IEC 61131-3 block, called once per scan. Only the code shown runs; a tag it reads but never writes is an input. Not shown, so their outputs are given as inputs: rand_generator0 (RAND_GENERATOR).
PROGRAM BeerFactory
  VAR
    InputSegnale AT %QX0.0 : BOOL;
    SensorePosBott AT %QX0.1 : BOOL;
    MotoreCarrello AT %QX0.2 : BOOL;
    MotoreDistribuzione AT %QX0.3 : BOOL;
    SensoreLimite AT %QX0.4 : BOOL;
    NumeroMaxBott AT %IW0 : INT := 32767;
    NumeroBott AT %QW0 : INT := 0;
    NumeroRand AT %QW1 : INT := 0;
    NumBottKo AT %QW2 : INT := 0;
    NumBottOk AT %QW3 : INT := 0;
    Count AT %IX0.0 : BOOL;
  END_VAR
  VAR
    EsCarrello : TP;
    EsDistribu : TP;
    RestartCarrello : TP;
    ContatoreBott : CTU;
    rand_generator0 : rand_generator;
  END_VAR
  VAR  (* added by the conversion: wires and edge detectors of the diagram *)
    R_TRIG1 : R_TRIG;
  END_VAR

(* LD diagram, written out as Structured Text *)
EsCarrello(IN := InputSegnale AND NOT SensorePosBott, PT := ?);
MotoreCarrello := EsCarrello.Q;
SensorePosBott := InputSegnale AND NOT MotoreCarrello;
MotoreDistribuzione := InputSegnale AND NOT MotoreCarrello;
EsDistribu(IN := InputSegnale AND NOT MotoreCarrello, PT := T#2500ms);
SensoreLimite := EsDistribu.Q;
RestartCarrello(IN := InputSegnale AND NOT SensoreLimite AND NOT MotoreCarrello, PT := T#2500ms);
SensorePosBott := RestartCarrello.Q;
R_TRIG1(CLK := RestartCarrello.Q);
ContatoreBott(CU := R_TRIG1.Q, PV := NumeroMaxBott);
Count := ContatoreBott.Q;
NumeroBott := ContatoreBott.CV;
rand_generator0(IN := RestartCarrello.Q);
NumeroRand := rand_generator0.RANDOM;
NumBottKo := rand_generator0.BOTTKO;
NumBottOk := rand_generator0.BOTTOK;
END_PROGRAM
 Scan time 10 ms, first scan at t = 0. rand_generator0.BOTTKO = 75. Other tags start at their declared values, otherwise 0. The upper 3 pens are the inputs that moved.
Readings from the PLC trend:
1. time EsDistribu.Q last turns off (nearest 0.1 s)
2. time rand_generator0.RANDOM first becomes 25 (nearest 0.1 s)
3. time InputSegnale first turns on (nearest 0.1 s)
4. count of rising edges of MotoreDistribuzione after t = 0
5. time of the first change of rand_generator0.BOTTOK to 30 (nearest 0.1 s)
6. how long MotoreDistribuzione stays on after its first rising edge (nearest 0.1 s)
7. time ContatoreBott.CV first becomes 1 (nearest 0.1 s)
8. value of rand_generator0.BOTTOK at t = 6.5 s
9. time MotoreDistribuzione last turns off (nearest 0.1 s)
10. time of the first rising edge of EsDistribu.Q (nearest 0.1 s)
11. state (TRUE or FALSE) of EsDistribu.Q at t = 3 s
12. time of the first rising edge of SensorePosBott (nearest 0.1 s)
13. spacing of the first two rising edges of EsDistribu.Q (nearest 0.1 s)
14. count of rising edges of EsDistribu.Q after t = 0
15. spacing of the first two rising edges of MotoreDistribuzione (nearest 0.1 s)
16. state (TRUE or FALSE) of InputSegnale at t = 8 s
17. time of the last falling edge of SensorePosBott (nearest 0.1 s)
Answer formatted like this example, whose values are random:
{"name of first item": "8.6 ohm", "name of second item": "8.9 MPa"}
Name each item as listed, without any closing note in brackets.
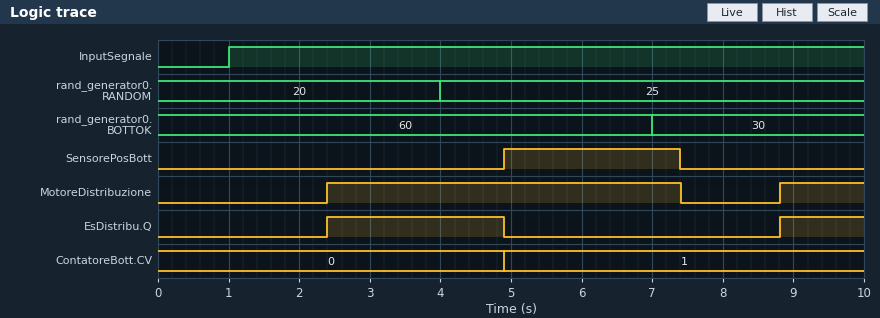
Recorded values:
{"time EsDistribu.Q last turns off": "4.9 s", "time rand_generator0.RANDOM first becomes 25": "4.0 s", "time InputSegnale first turns on": "1.0 s", "count of rising edges of MotoreDistribuzione after t = 0": "2", "time of the first change of rand_generator0.BOTTOK to 30": "7.0 s", "how long MotoreDistribuzione stays on after its first rising edge": "5.0 s", "time ContatoreBott.CV first becomes 1": "4.9 s", "value of rand_generator0.BOTTOK at t = 6.5 s": "60", "time MotoreDistribuzione last turns off": "7.4 s", "time of the first rising edge of EsDistribu.Q": "2.4 s", "state (TRUE or FALSE) of EsDistribu.Q at t = 3 s": "TRUE", "time of the first rising edge of SensorePosBott": "4.9 s", "spacing of the first two rising edges of EsDistribu.Q": "6.4 s", "count of rising edges of EsDistribu.Q after t = 0": "2", "spacing of the first two rising edges of MotoreDistribuzione": "6.4 s", "state (TRUE or FALSE) of InputSegnale at t = 8 s": "TRUE", "time of the last falling edge of SensorePosBott": "7.4 s"}
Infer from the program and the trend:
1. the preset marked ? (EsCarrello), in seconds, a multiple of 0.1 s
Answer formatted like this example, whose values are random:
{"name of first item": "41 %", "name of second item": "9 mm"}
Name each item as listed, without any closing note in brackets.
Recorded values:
{"the preset marked ? (EsCarrello), in seconds, a multiple of 0.1 s": "1.4 s"}
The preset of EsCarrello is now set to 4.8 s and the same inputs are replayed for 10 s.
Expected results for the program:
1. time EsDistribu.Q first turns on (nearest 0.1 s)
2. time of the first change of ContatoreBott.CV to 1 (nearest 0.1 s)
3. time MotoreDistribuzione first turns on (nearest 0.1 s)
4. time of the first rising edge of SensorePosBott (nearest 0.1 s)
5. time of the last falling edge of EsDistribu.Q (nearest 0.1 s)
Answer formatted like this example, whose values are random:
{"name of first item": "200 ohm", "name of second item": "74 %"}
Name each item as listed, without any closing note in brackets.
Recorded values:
{"time EsDistribu.Q first turns on": "5.8 s", "time of the first change of ContatoreBott.CV to 1": "8.3 s", "time MotoreDistribuzione first turns on": "5.8 s", "time of the first rising edge of SensorePosBott": "8.3 s", "time of the last falling edge of EsDistribu.Q": "8.3 s"}
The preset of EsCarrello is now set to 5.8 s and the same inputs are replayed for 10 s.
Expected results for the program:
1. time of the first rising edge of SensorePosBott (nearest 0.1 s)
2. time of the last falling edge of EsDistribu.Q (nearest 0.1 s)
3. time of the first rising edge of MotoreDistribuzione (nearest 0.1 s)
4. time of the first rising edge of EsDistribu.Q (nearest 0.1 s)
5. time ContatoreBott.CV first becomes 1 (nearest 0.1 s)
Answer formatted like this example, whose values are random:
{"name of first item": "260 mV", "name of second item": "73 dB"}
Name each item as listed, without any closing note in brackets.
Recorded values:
{"time of the first rising edge of SensorePosBott": "9.3 s", "time of the last falling edge of EsDistribu.Q": "9.3 s", "time of the first rising edge of MotoreDistribuzione": "6.8 s", "time of the first rising edge of EsDistribu.Q": "6.8 s", "time ContatoreBott.CV first becomes 1": "9.3 s"}
